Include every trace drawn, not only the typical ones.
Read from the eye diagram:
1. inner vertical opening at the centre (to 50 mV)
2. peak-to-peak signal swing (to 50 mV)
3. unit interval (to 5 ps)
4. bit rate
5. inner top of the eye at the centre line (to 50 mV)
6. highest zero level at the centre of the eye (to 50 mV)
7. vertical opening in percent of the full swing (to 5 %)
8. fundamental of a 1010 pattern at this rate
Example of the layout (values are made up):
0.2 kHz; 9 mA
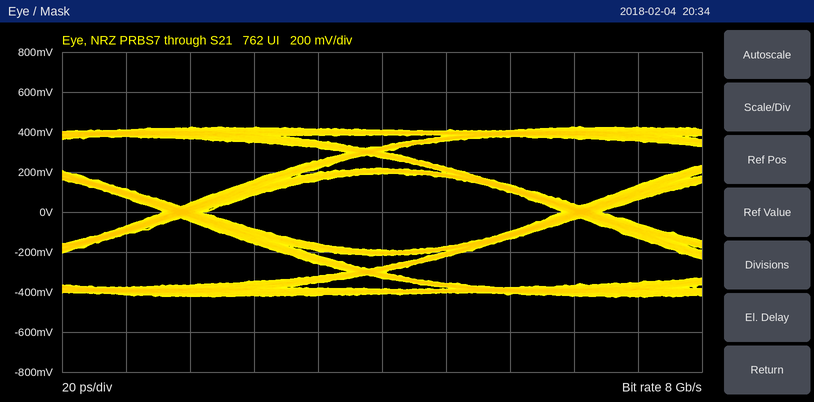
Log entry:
400 mV; 850 mV; 125 ps; 8 Gb/s; 200 mV; -200 mV; 45 %; 4 GHz
